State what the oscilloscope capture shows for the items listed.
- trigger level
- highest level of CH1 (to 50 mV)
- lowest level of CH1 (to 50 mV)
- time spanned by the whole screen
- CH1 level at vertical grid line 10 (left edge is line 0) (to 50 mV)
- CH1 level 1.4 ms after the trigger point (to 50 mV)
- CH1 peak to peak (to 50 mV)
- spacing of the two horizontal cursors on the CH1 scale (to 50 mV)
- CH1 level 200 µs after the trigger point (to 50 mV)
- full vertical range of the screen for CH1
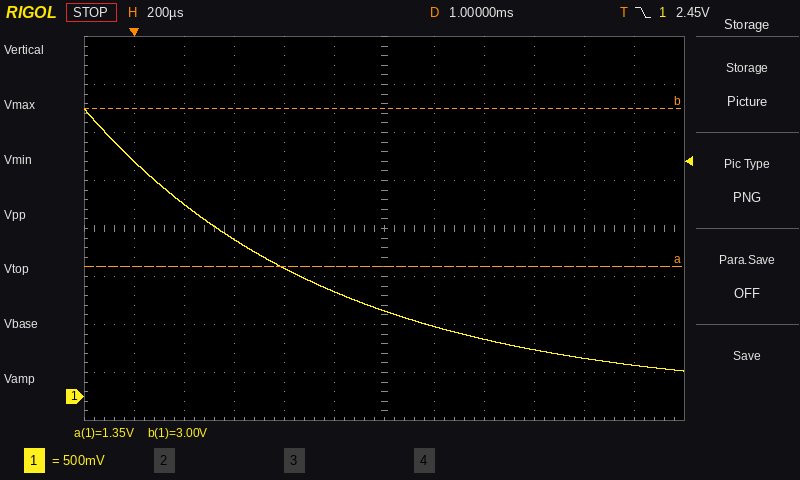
2.45 V
3.00 V
250 mV
2.4 ms
400 mV
600 mV
2.75 V
1.65 V
2.00 V
4 V
